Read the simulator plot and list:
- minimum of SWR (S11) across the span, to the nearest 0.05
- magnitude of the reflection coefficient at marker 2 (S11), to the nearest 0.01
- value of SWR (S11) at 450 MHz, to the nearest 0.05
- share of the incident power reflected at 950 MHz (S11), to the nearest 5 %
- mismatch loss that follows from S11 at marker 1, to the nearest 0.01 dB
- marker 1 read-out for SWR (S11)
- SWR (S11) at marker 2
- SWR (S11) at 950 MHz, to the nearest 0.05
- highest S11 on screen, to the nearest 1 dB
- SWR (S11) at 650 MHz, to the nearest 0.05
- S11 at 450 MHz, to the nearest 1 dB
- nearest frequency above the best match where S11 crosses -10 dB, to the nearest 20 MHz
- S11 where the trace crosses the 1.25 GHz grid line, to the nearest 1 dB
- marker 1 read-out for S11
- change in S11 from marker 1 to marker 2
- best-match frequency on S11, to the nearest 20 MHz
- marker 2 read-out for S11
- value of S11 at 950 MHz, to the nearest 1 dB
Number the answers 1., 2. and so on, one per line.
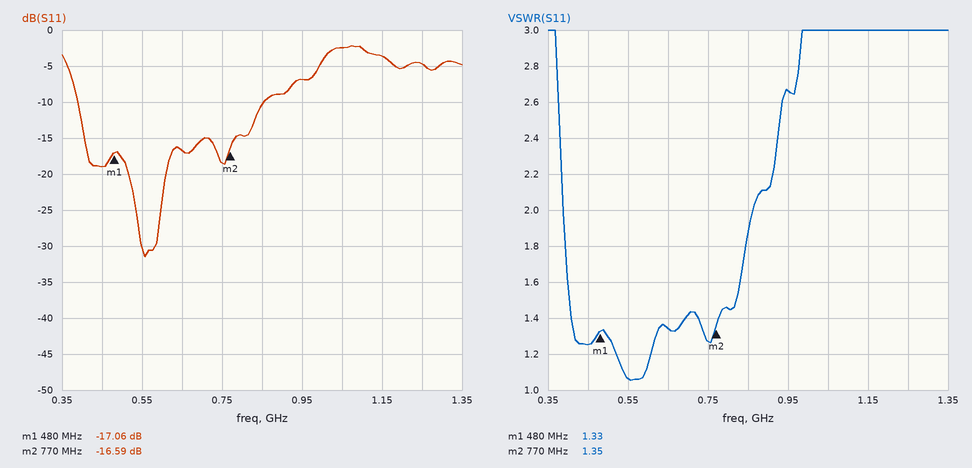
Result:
1. 1.05
2. 0.15
3. 1.25
4. 20 %
5. 0.09 dB
6. 1.33
7. 1.35
8. 2.65
9. -2 dB
10. 1.35
11. -19 dB
12. 860 MHz
13. -5 dB
14. -17.06 dB
15. 0.47 dB
16. 560 MHz
17. -16.59 dB
18. -7 dB
